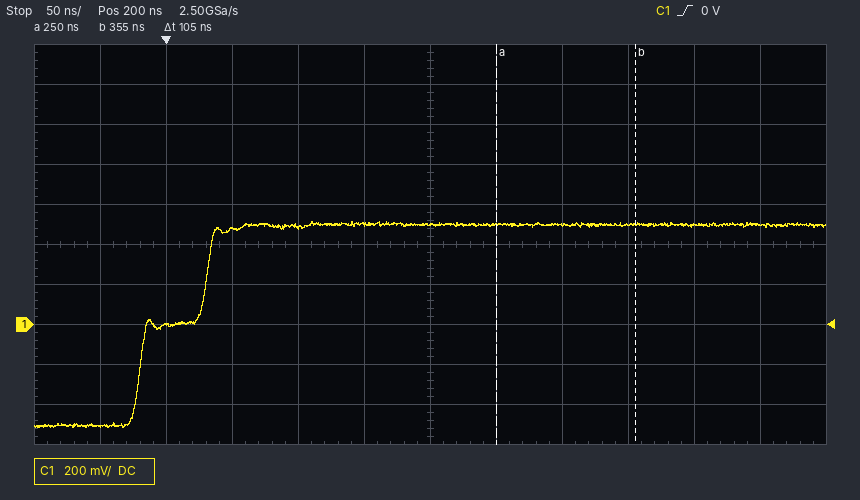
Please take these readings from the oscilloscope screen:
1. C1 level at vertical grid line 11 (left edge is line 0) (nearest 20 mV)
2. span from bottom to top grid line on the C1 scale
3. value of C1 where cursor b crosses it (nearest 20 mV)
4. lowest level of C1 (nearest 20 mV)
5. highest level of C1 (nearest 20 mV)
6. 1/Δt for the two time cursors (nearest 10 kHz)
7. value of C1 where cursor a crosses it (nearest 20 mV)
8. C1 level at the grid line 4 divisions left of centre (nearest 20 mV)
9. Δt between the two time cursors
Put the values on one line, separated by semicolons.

500 mV; 2 V; 500 mV; -520 mV; 520 mV; 9.52 MHz; 500 mV; 0 mV; 105 ns
